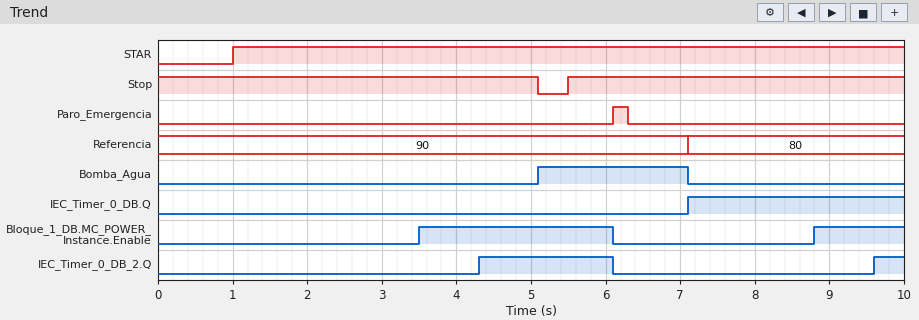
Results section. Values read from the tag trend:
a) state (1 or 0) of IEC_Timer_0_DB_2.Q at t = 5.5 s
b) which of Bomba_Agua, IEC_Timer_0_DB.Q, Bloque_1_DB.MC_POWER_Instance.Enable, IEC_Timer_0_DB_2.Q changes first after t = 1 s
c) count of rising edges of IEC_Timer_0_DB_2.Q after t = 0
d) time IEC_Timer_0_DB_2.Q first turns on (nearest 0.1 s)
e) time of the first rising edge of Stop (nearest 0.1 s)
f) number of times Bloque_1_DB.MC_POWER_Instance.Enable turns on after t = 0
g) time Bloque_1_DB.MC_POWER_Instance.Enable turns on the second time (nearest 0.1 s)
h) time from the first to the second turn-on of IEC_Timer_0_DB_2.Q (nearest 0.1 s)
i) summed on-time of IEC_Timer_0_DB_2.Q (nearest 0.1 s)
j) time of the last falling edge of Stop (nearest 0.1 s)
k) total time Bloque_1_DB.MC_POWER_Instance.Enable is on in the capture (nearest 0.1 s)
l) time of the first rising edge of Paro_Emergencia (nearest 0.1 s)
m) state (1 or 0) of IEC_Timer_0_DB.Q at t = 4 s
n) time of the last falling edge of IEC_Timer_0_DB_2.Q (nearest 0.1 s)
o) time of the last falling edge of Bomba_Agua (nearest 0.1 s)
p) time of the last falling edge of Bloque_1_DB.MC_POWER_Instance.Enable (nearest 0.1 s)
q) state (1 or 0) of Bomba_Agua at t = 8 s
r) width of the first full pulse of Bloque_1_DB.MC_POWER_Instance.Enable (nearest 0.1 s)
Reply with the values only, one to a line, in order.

1
Bloque_1_DB.MC_POWER_Instance.Enable
2
4.3 s
5.5 s
2
8.8 s
5.3 s
2.2 s
5.1 s
3.8 s
6.1 s
0
6.1 s
7.1 s
6.1 s
0
2.6 s
